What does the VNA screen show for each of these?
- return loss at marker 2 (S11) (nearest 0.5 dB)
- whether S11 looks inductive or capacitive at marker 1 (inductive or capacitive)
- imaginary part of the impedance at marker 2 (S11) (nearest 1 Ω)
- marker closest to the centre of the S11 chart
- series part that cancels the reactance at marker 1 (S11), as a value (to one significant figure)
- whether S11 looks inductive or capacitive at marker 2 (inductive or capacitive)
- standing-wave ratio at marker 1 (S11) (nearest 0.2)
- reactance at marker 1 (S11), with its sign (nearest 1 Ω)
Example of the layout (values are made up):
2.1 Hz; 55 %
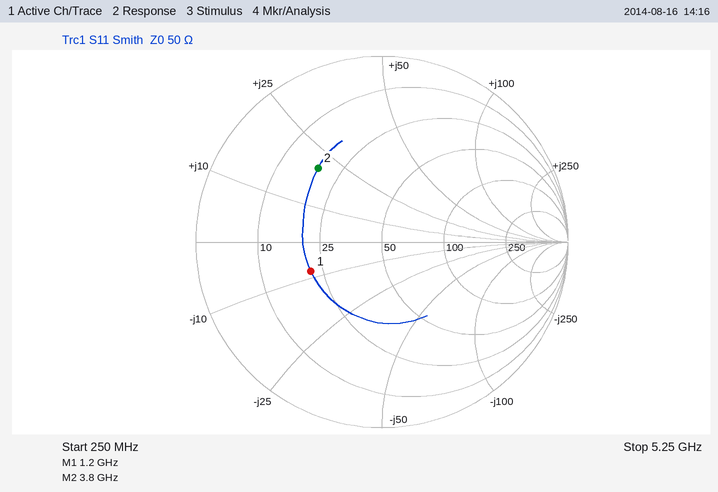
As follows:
5.5 dB; capacitive; +20 Ω; marker 1; 1 nH; inductive; 2.4; -8 Ω
